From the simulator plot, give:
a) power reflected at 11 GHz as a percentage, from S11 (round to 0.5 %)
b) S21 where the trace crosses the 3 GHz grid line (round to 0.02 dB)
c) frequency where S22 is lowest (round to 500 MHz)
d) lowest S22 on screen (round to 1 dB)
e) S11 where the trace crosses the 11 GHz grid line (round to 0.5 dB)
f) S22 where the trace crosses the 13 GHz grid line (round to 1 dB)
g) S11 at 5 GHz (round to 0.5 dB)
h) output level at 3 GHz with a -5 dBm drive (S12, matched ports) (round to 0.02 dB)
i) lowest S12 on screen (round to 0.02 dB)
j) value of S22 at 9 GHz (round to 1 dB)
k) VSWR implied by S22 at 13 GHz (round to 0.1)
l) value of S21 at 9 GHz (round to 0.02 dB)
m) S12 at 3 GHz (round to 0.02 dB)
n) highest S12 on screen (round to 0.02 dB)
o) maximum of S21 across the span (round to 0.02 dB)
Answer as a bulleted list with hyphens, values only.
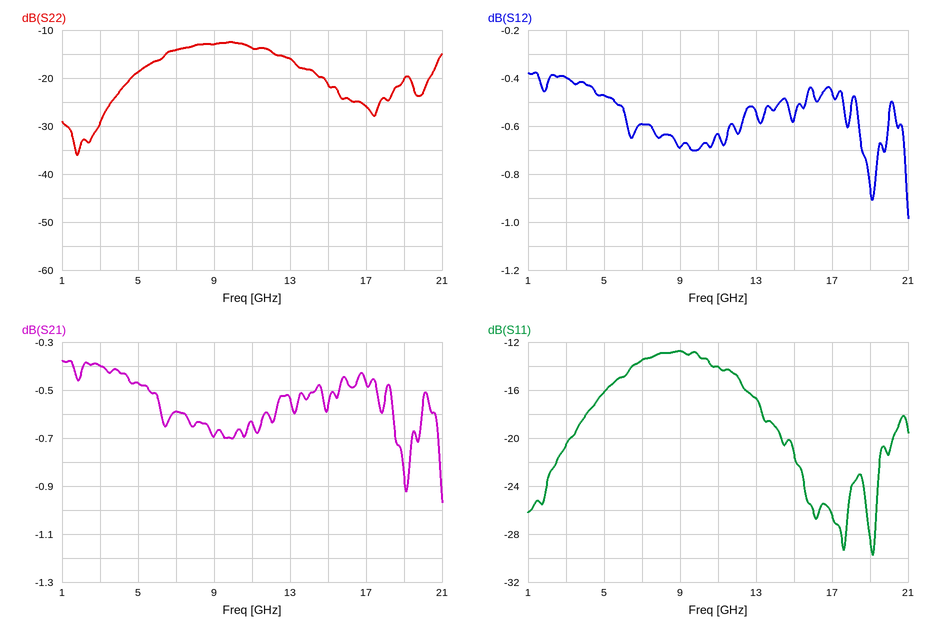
- 4.0 %
- -0.40 dB
- 2.0 GHz
- -36 dB
- -14.0 dB
- -16 dB
- -16.0 dB
- -5.40 dBm
- -0.98 dB
- -13 dB
- 1.4
- -0.70 dB
- -0.40 dB
- -0.38 dB
- -0.38 dB
